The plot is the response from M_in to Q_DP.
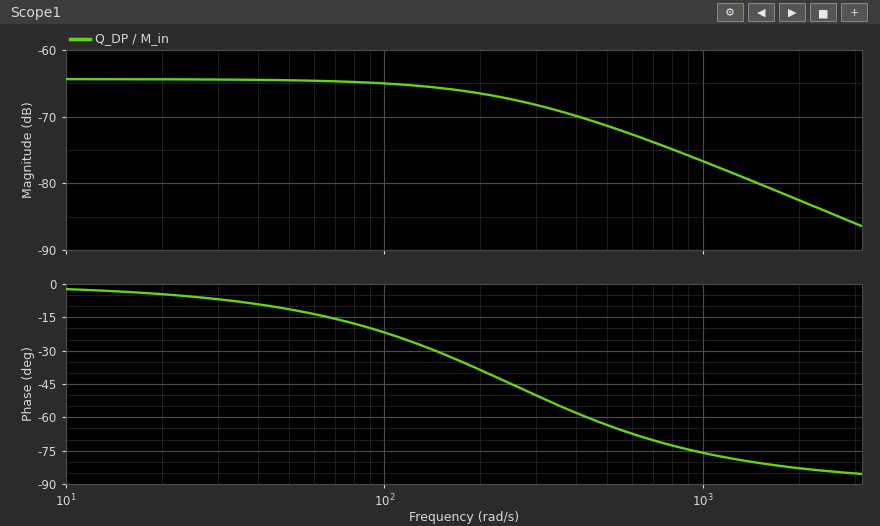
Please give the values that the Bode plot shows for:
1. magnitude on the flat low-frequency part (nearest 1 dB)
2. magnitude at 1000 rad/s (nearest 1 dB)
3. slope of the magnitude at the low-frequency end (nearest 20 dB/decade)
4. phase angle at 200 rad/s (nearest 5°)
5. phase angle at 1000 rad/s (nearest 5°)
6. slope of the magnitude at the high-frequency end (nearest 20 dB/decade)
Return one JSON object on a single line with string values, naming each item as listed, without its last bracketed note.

{"magnitude on the flat low-frequency part": "-64 dB", "magnitude at 1000 rad/s": "-77 dB", "slope of the magnitude at the low-frequency end": "0 dB/decade", "phase angle at 200 rad/s": "-40°", "phase angle at 1000 rad/s": "-75°", "slope of the magnitude at the high-frequency end": "-20 dB/decade"}
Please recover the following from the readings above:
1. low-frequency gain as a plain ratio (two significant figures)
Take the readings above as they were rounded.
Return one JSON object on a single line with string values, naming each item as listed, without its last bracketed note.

{"low-frequency gain as a plain ratio": "0.00063"}
